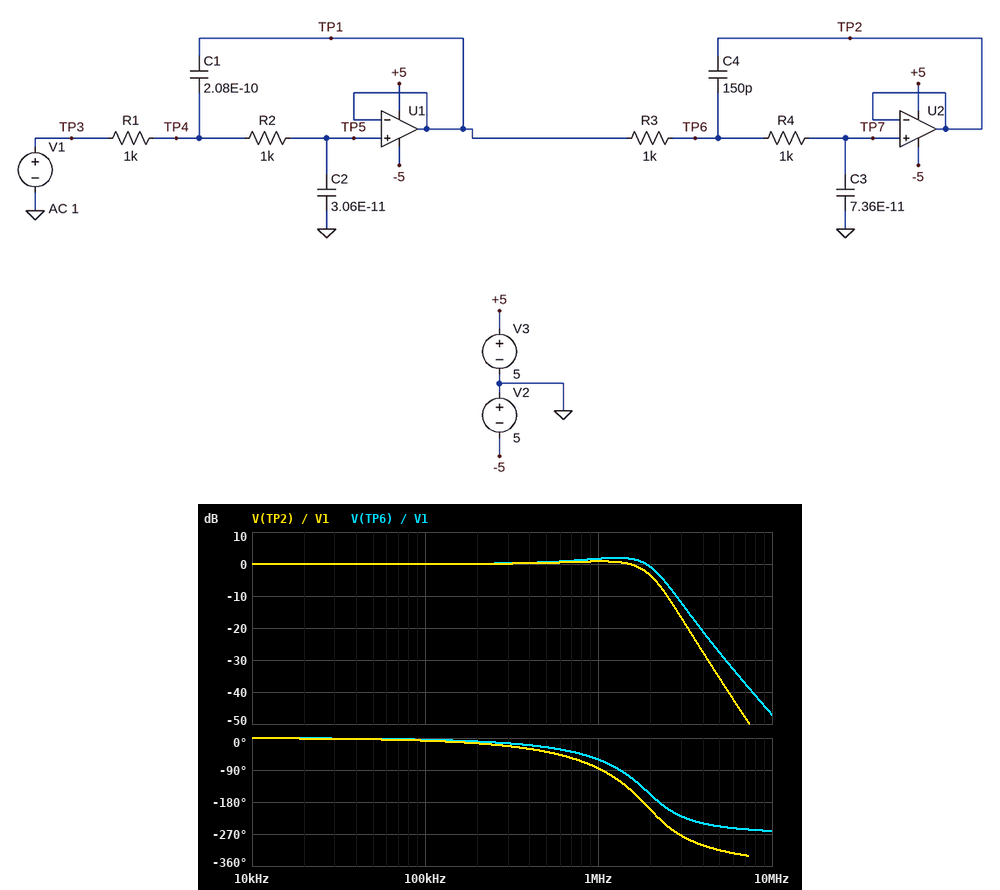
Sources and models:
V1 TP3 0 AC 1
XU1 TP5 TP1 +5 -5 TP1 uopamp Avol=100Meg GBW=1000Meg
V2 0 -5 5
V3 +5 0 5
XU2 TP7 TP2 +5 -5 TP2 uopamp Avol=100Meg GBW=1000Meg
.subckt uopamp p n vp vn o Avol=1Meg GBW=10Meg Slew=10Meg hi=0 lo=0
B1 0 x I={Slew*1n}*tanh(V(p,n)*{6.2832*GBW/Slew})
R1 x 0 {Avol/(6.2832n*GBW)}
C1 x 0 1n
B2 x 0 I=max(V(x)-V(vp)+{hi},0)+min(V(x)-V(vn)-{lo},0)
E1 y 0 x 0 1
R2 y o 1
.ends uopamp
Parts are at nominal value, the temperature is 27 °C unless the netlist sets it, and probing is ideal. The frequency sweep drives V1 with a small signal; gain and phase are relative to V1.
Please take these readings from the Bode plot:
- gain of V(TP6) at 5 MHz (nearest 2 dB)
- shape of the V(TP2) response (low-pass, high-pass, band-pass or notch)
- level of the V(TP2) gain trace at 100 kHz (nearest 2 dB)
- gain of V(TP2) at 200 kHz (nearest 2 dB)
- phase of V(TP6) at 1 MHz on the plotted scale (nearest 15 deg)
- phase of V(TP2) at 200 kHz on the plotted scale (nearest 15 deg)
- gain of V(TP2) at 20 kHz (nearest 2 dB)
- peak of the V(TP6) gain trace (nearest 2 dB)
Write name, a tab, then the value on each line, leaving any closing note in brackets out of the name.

gain of V(TP6) at 5 MHz	-28 dB
shape of the V(TP2) response	low-pass
level of the V(TP2) gain trace at 100 kHz	0 dB
gain of V(TP2) at 200 kHz	0 dB
phase of V(TP6) at 1 MHz on the plotted scale	-60 deg
phase of V(TP2) at 200 kHz on the plotted scale	-15 deg
gain of V(TP2) at 20 kHz	0 dB
peak of the V(TP6) gain trace	2 dB
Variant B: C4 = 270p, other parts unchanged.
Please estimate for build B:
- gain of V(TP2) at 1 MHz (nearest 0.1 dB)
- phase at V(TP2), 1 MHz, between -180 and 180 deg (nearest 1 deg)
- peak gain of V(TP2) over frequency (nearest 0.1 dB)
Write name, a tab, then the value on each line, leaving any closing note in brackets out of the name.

gain of V(TP2) at 1 MHz	2.0 dB
phase at V(TP2), 1 MHz, between -180 and 180 deg	-104 deg
peak gain of V(TP2) over frequency	2.1 dB
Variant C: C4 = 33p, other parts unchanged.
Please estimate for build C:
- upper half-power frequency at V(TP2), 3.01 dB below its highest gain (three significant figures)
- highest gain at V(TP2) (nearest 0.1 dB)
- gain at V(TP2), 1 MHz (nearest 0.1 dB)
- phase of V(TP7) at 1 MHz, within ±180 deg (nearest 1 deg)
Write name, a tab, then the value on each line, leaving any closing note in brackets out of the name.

upper half-power frequency at V(TP2), 3.01 dB below its highest gain	1.93 MHz
highest gain at V(TP2)	0 dB
gain at V(TP2), 1 MHz	-0.7 dB
phase of V(TP7) at 1 MHz, within ±180 deg	-73 deg
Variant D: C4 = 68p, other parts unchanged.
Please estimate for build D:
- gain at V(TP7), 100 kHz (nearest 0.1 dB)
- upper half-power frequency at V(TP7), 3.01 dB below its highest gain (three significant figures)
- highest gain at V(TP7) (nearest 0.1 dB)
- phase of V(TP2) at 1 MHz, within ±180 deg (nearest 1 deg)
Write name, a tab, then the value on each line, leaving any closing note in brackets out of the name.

gain at V(TP7), 100 kHz	0 dB
upper half-power frequency at V(TP7), 3.01 dB below its highest gain	1.99 MHz
highest gain at V(TP7)	0 dB
phase of V(TP2) at 1 MHz, within ±180 deg	-76 deg
